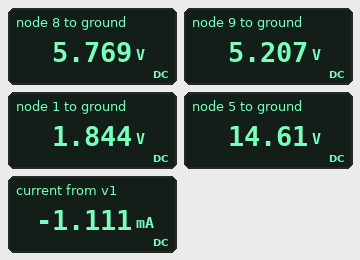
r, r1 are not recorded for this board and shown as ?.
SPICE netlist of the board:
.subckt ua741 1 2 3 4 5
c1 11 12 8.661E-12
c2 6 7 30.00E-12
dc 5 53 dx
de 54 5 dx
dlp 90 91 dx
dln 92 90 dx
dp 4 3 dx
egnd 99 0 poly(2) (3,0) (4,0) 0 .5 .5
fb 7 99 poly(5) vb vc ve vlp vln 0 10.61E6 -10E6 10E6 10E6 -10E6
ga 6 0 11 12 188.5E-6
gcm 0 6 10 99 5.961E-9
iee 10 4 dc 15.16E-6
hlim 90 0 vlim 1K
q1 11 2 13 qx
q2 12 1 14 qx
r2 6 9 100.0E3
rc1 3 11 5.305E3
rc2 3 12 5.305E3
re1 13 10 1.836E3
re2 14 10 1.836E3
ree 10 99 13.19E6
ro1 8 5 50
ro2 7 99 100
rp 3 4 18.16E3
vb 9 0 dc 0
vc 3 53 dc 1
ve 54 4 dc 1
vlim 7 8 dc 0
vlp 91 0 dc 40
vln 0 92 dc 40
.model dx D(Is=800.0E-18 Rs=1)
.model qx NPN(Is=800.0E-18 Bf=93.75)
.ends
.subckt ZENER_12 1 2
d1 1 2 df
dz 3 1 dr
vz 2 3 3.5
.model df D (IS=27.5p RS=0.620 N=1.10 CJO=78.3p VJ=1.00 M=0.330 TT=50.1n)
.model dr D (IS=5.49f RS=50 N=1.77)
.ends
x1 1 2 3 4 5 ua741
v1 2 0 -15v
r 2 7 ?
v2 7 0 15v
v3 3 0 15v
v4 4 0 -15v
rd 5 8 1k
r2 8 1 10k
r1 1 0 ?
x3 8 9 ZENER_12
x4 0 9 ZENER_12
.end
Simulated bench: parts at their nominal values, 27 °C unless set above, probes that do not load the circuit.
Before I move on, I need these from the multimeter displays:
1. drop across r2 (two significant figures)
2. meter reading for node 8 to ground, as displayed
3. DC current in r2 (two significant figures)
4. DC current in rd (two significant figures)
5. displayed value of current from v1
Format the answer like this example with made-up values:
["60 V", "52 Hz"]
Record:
["3.9 V", "5.769 V", "390 µA", "8.8 mA", "-1.111 mA"]
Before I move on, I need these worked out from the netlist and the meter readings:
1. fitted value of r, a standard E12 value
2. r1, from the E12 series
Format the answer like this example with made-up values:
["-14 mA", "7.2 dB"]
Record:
["27 kΩ", "4.7 kΩ"]
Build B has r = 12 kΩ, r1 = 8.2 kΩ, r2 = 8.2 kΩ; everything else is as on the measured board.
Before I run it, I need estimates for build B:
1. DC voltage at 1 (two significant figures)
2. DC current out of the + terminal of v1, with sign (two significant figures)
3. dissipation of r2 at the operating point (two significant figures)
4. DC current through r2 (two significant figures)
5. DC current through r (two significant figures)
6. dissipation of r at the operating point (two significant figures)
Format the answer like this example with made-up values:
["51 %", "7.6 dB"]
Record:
["2.9 V", "-2.5 mA", "1.0 mW", "350 µA", "2.5 mA", "75 mW"]
